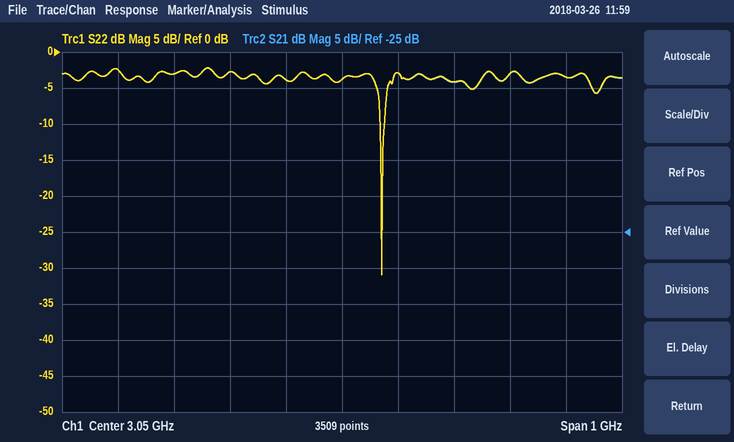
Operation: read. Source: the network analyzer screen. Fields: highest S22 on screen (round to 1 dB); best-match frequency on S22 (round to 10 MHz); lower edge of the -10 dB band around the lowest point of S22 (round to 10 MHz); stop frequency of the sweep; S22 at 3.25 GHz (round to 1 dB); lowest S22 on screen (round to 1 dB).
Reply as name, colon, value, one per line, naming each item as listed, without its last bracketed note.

highest S22 on screen: -2 dB
best-match frequency on S22: 3.12 GHz
lower edge of the -10 dB band around the lowest point of S22: 3.12 GHz
stop frequency of the sweep: 3.55 GHz
S22 at 3.25 GHz: -4 dB
lowest S22 on screen: -31 dB
